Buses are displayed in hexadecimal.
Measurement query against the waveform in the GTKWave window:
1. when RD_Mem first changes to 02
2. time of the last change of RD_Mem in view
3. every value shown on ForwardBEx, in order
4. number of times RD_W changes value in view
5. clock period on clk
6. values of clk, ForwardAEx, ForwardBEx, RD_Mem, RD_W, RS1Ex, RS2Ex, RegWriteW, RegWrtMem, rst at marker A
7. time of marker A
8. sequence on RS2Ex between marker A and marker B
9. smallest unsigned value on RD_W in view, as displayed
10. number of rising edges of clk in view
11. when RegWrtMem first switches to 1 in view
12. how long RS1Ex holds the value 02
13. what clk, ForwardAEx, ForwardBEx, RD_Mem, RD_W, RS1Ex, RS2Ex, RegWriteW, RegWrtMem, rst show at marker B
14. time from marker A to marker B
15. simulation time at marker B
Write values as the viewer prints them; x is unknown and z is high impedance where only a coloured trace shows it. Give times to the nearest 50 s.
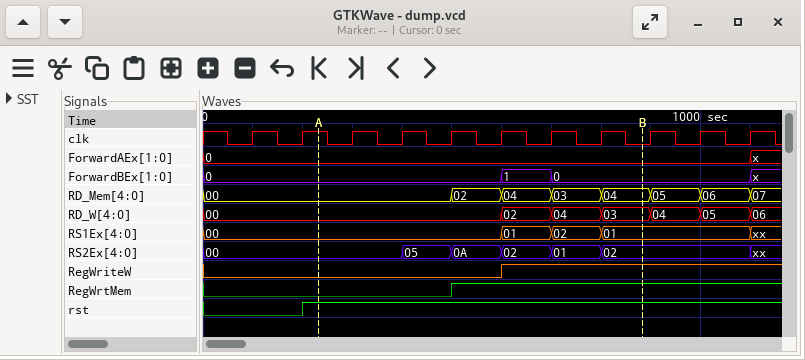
500 s
1100 s
0, 1, 0, x
6
100 s
clk=1, ForwardAEx=0, ForwardBEx=0, RD_Mem=00, RD_W=00, RS1Ex=00, RS2Ex=00, RegWriteW=0, RegWrtMem=0, rst=1
250 s
00, 05, 0A, 02, 01, 02
00
11
500 s
100 s
clk=0, ForwardAEx=0, ForwardBEx=0, RD_Mem=04, RD_W=03, RS1Ex=01, RS2Ex=02, RegWriteW=1, RegWrtMem=1, rst=1
650 s
900 s
